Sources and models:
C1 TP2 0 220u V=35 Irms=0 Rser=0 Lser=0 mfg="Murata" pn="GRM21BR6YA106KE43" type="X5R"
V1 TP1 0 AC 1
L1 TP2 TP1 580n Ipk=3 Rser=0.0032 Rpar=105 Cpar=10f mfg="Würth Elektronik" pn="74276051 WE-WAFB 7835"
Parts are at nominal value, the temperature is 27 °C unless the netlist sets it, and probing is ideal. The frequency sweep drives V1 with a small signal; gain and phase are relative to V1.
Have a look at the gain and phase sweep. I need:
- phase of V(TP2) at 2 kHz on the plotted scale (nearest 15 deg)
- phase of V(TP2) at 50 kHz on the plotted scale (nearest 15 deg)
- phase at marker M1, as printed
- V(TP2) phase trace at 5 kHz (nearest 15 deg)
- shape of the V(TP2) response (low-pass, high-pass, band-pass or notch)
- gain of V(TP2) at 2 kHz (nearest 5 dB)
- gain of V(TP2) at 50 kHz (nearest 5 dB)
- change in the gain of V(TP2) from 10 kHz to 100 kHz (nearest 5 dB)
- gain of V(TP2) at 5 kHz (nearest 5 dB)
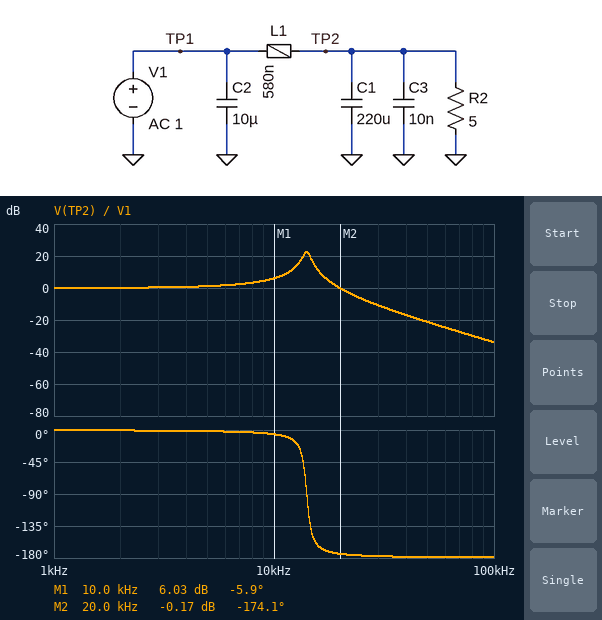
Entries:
0 deg
-180 deg
-5.9 deg
0 deg
low-pass
0 dB
-20 dB
-40 dB
0 dB
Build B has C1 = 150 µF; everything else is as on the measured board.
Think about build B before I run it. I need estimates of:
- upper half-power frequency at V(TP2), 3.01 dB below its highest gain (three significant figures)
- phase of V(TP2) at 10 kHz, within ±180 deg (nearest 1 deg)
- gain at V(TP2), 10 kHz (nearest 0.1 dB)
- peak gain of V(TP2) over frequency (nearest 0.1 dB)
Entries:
17.6 kHz
-3 deg
3.6 dB
23.8 dB
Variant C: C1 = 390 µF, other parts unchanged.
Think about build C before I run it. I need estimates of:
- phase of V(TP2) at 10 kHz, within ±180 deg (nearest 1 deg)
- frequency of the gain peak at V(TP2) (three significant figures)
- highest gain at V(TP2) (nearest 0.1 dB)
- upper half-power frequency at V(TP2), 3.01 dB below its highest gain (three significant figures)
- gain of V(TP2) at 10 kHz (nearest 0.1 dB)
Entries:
-39 deg
10.6 kHz
20.8 dB
11.0 kHz
17.2 dB
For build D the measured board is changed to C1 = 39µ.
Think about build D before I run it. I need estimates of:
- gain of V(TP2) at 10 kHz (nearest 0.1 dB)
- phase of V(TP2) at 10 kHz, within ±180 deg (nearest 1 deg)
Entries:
0.8 dB
-1 deg
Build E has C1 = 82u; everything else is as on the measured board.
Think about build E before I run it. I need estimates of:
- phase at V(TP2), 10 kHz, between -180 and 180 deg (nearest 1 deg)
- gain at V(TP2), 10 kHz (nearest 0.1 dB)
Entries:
-2 deg
1.8 dB
